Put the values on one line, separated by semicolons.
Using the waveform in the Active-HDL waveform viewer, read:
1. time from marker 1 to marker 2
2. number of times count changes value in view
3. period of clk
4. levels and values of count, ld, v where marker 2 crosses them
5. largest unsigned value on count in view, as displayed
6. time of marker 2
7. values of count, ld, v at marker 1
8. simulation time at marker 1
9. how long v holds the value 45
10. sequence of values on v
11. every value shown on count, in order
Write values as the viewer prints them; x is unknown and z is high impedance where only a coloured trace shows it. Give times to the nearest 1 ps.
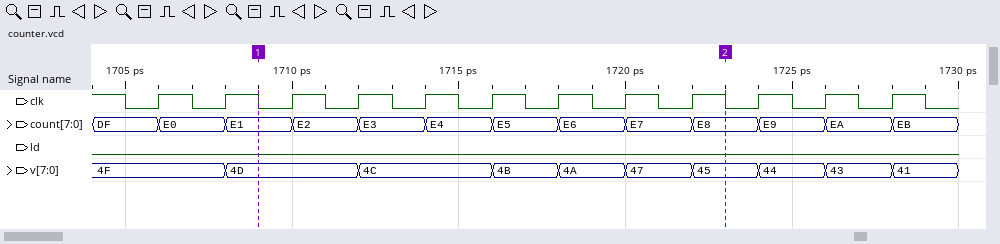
14 ps; 12; 2 ps; count=E8, ld=0, v=45; EB; 1723 ps; count=E1, ld=0, v=4D; 1709 ps; 2 ps; 4F, 4D, 4C, 4B, 4A, 47, 45, 44, 43, 41; DF, E0, E1, E2, E3, E4, E5, E6, E7, E8, E9, EA, EB
